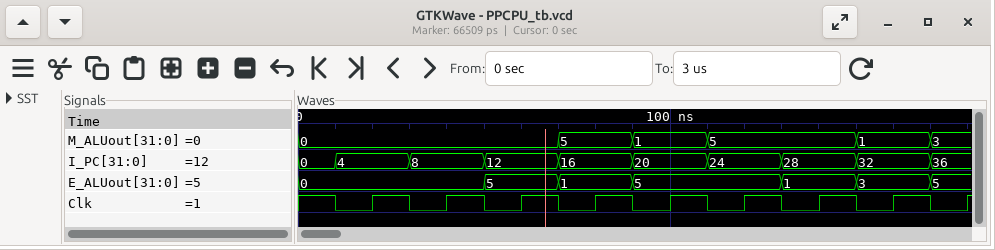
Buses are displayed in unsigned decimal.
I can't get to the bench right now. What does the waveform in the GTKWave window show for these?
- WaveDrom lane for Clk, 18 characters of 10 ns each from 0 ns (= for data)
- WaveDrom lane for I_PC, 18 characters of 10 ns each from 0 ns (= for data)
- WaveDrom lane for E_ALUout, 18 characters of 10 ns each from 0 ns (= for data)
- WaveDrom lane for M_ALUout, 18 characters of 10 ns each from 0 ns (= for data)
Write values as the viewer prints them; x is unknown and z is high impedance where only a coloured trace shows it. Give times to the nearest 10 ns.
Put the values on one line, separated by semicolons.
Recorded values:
{name: 'Clk', wave: '101010101010101010'}; {name: 'I_PC', wave: '==.=.=.=.=.=.=.=.=', data: '0 4 8 12 16 20 24 28 32 36'}; {name: 'E_ALUout', wave: '=....=.=.=...=.=.=', data: '0 5 1 5 1 3 5'}; {name: 'M_ALUout', wave: '=......=.=.=...=.=', data: '0 5 1 5 1 3'}
